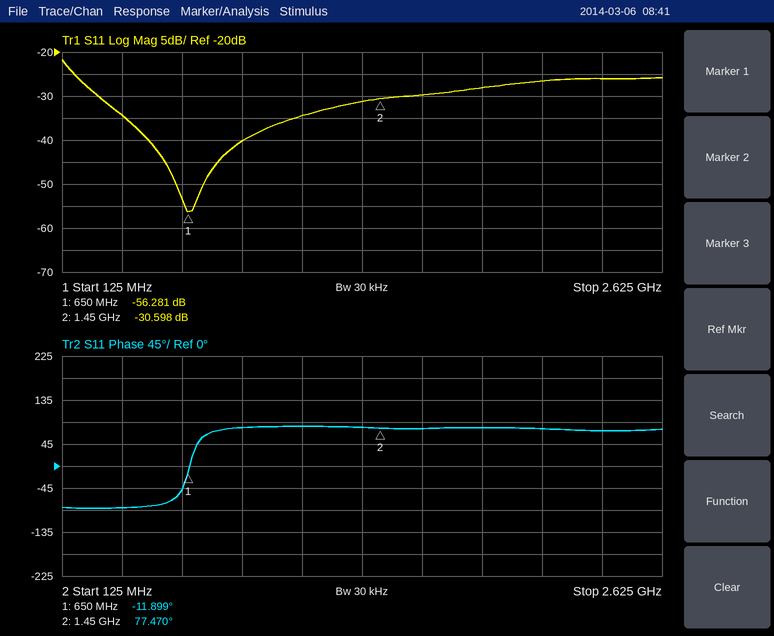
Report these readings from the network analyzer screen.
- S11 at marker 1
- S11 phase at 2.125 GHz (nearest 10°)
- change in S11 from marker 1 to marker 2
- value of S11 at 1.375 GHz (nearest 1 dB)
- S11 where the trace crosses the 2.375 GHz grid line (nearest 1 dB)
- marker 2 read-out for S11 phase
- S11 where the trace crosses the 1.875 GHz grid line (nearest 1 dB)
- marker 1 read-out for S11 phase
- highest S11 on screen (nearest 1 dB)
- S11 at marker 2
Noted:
-56.281 dB
80°
25.683 dB
-31 dB
-26 dB
77.470°
-28 dB
-11.899°
-22 dB
-30.598 dB
